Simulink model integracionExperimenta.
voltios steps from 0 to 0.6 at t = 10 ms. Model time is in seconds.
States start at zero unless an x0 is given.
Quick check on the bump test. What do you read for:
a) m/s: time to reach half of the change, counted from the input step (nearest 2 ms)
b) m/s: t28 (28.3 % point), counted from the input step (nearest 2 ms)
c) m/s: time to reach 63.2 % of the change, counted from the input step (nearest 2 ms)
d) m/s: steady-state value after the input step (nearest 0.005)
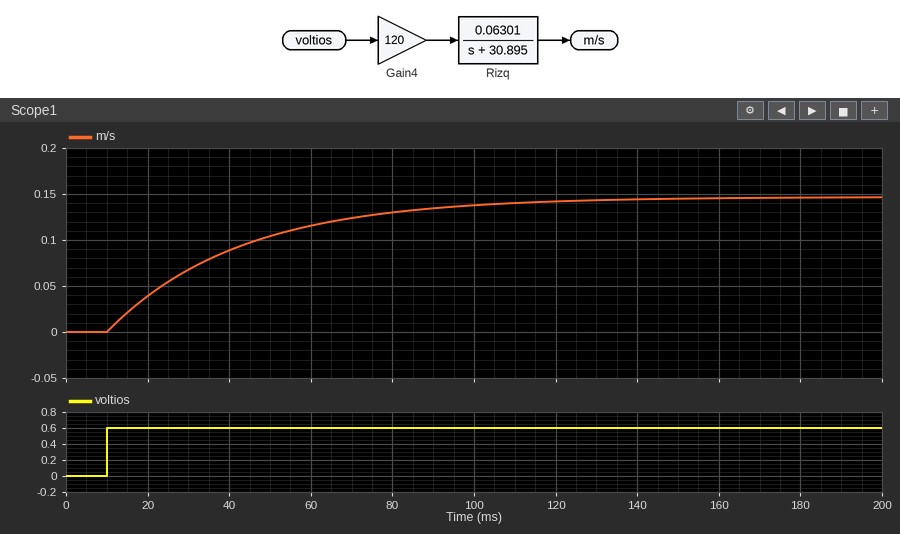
22 ms
10 ms
32 ms
0.145
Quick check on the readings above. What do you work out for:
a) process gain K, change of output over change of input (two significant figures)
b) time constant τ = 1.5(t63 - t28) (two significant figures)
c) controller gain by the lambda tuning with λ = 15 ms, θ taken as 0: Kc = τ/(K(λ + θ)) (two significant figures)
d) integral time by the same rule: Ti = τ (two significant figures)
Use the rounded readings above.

0.24
33 ms
9.2
33 ms
